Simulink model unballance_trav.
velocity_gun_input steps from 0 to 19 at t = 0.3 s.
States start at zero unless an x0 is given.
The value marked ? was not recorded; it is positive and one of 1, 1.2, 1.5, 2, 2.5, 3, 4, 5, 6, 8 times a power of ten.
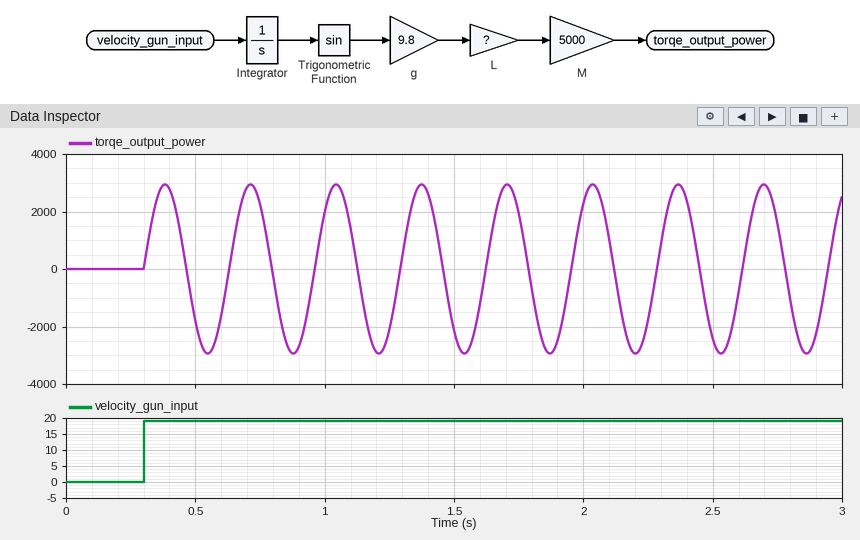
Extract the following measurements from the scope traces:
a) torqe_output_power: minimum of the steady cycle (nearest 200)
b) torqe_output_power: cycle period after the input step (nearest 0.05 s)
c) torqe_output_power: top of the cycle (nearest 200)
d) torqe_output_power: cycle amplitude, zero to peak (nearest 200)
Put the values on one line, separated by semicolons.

-3000; 0.35 s; 3000; 3000
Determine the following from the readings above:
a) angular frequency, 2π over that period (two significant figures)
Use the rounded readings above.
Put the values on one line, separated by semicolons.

18 rad/s
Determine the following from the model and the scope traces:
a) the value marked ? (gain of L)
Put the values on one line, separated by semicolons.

0.06
